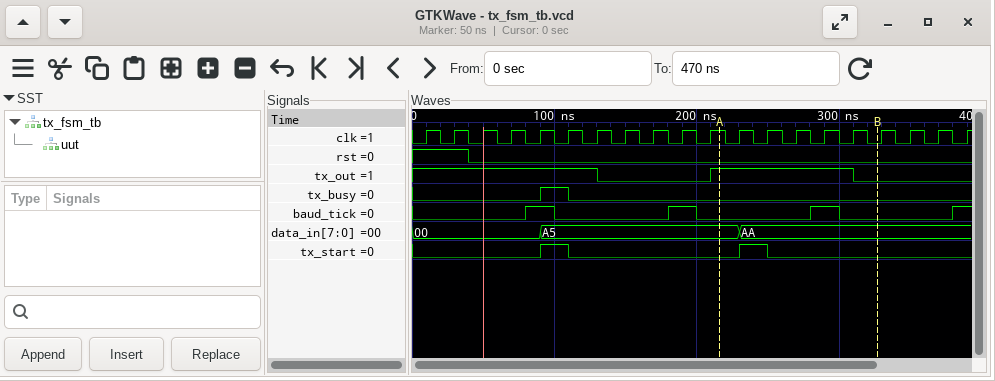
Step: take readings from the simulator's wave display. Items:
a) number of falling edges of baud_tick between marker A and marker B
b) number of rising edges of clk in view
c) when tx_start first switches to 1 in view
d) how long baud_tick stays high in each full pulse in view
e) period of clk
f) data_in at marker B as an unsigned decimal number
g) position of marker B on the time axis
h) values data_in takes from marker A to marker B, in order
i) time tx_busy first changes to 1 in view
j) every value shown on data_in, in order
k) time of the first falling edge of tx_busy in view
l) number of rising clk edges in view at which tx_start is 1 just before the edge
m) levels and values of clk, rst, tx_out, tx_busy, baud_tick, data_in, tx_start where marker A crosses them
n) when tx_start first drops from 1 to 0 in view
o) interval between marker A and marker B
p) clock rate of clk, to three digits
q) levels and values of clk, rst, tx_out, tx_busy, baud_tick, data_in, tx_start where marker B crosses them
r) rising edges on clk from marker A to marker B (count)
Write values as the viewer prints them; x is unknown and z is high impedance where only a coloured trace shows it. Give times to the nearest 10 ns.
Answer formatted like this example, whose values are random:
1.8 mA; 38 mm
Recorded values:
1; 20; 90 ns; 20 ns, 20 ns, 20 ns; 20 ns; 170; 330 ns; A5, AA; 90 ns; 00, A5, AA; 110 ns; 2; clk=1, rst=0, tx_out=1, tx_busy=0, baud_tick=0, data_in=A5, tx_start=0; 110 ns; 110 ns; 50.0 MHz; clk=0, rst=0, tx_out=0, tx_busy=0, baud_tick=0, data_in=AA, tx_start=0; 5
